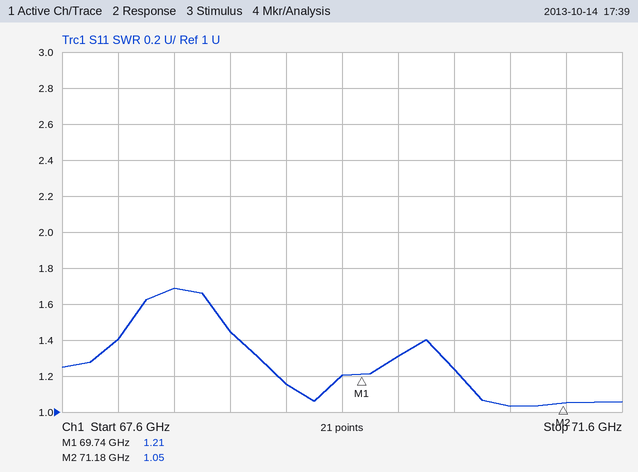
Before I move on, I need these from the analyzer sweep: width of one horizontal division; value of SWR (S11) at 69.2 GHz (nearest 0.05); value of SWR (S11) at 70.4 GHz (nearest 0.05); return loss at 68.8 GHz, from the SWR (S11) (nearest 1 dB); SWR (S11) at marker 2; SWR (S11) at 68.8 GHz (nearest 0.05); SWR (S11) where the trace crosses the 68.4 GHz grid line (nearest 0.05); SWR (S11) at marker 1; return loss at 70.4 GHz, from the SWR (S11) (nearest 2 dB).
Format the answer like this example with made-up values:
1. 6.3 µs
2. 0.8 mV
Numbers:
1. 400 MHz
2. 1.15
3. 1.25
4. 15 dB
5. 1.05
6. 1.45
7. 1.70
8. 1.21
9. 20 dB
